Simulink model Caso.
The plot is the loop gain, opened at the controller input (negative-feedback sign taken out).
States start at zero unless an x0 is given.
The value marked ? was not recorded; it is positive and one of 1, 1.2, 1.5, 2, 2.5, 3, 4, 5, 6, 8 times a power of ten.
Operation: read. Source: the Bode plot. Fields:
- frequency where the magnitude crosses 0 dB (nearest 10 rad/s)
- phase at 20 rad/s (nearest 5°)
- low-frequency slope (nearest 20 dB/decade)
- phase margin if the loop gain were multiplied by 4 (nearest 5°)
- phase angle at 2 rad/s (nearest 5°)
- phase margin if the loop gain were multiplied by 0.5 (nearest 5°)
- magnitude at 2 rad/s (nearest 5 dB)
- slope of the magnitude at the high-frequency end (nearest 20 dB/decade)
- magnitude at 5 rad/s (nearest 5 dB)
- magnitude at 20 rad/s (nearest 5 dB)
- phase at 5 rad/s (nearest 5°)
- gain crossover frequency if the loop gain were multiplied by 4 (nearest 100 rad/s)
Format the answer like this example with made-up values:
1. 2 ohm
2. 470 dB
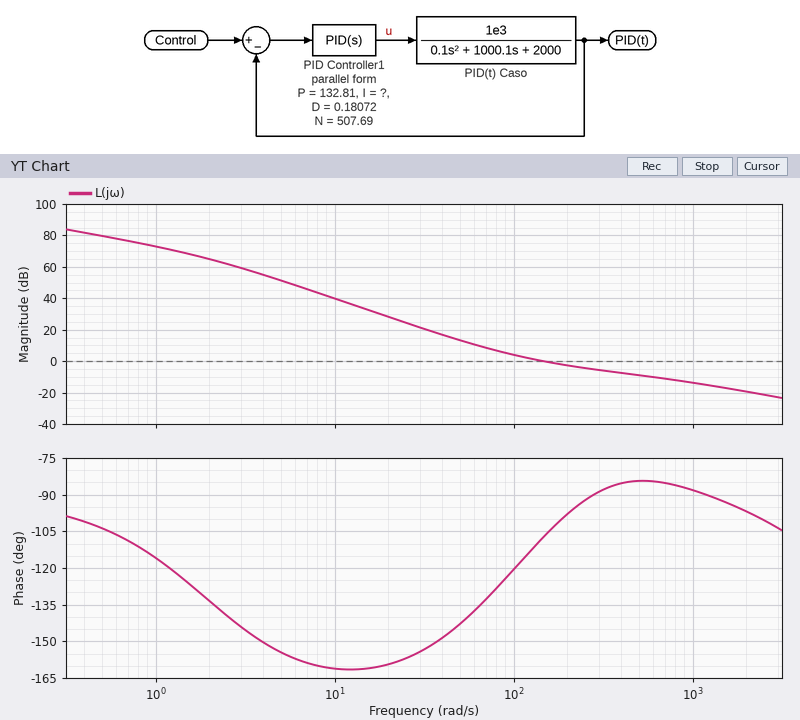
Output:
1. 150 rad/s
2. -160°
3. -20 dB/decade
4. 95°
5. -135°
6. 55°
7. 65 dB
8. -20 dB/decade
9. 50 dB
10. 30 dB
11. -155°
12. 800 rad/s
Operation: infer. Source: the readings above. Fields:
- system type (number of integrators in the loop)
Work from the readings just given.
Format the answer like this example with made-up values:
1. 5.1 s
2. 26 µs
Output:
1. 1
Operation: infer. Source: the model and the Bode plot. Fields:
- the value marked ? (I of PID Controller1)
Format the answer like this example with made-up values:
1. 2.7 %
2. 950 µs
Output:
1. 10000
